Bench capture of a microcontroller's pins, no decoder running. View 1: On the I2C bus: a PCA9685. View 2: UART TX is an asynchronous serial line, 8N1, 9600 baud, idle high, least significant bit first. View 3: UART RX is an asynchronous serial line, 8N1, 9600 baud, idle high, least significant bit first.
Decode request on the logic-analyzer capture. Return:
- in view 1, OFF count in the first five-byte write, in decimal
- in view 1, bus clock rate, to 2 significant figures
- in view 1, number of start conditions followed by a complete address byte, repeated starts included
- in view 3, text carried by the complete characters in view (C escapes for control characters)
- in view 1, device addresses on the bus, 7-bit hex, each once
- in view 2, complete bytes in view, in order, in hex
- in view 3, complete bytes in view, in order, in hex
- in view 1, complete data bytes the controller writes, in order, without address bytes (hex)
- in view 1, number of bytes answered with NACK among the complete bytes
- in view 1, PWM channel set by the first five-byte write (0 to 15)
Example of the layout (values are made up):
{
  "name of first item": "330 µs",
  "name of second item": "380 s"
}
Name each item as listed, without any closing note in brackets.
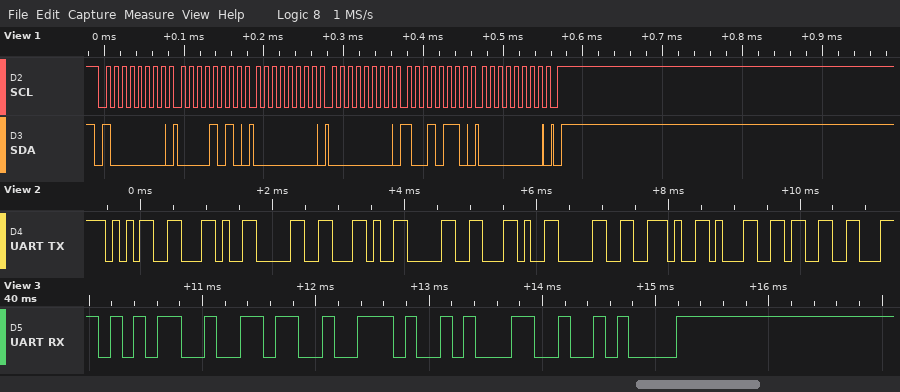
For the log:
{
  "in view 1, OFF count in the first five-byte write, in decimal": "150",
  "in view 1, bus clock rate, to 2 significant figures": "100 kHz",
  "in view 1, number of start conditions followed by a complete address byte, repeated starts included": "1",
  "in view 3, text carried by the complete characters in view": "\"56.1\\n\"",
  "in view 1, device addresses on the bus, 7-bit hex, each once": "0x40",
  "in view 2, complete bytes in view, in order, in hex": "35 2C 30 2C 30 2C 30 2E 31 33",
  "in view 3, complete bytes in view, in order, in hex": "35 36 2E 31 0A",
  "in view 1, complete data bytes the controller writes, in order, without address bytes": "0A 00 00 96 00",
  "in view 1, number of bytes answered with NACK among the complete bytes": "0",
  "in view 1, PWM channel set by the first five-byte write": "1"
}
